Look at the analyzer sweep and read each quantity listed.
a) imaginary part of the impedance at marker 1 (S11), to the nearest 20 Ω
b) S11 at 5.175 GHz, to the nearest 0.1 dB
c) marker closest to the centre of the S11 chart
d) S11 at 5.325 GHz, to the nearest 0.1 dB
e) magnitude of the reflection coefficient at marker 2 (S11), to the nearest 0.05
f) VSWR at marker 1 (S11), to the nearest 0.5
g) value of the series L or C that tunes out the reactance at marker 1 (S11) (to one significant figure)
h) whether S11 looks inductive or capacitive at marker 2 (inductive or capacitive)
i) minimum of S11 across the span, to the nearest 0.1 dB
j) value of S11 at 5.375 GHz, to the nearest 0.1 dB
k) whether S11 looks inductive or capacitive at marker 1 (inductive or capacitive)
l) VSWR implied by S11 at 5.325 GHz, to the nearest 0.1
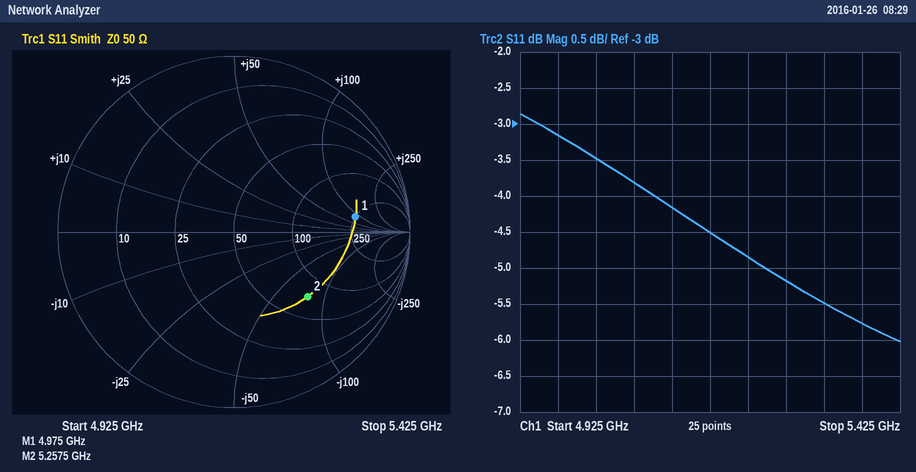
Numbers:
+80 Ω
-4.5 dB
marker 2
-5.5 dB
0.55
5.5
400 fF
capacitive
-6.0 dB
-5.8 dB
inductive
3.3
